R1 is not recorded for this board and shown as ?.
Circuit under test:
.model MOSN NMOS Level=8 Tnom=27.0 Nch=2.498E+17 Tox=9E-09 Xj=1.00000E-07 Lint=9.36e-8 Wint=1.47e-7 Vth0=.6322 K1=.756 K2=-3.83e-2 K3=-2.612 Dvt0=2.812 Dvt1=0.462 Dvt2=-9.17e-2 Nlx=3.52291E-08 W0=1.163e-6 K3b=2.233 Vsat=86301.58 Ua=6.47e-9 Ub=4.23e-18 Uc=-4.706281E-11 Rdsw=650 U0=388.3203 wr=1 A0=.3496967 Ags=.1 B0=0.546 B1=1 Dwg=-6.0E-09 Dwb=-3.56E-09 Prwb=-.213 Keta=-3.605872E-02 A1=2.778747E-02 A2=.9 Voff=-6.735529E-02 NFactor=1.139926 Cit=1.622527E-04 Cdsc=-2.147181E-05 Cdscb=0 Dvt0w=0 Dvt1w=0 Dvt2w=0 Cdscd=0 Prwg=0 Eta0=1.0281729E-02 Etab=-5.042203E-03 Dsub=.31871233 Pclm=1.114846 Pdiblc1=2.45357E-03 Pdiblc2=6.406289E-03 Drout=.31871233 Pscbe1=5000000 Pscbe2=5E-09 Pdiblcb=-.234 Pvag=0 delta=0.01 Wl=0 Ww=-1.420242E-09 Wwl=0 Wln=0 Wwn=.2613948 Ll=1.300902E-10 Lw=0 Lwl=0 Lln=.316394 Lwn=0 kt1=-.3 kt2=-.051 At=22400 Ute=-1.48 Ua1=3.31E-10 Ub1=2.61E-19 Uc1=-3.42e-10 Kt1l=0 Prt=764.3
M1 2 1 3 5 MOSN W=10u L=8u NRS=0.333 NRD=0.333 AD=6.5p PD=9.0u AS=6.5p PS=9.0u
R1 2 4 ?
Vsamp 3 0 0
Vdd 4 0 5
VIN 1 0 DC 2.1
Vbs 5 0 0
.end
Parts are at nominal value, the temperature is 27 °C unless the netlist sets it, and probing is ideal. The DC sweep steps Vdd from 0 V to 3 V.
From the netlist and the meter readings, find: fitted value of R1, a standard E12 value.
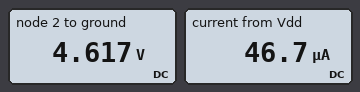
8.2 kΩ
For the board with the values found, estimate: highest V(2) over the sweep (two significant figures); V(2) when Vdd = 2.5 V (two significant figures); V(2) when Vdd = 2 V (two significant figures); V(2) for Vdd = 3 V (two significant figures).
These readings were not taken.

2.6 V
2.1 V
1.6 V
2.6 V
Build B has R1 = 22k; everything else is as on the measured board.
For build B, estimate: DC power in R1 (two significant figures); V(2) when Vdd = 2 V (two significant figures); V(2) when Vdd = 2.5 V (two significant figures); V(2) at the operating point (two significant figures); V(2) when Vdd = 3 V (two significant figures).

48 µW
1.0 V
1.5 V
4.0 V
2.0 V
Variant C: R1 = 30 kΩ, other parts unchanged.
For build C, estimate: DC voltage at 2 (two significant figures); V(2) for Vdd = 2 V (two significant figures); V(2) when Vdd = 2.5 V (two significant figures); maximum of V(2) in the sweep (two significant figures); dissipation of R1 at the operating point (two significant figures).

3.6 V
780 mV
1.1 V
1.6 V
65 µW
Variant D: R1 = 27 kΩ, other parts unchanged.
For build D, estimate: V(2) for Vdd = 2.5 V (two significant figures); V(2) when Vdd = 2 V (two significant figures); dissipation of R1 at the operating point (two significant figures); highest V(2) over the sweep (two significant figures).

1.3 V
850 mV
58 µW
1.8 V
